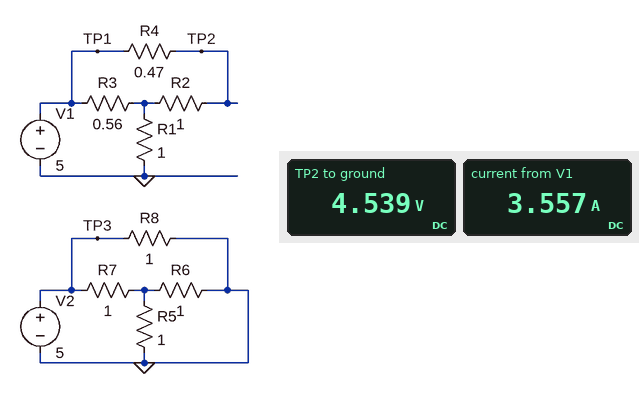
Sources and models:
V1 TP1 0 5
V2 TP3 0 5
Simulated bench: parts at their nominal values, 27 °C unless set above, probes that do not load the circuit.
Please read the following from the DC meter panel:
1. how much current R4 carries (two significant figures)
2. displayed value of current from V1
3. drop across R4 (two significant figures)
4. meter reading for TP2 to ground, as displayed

980 mA
3.557 A
460 mV
4.539 V
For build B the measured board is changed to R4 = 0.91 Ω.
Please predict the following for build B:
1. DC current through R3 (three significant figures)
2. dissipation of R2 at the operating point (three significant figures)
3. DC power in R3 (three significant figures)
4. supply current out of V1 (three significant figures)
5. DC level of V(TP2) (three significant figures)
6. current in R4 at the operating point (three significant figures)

2.70 A
626 mW
4.08 W
3.49 A
4.28 V
791 mA
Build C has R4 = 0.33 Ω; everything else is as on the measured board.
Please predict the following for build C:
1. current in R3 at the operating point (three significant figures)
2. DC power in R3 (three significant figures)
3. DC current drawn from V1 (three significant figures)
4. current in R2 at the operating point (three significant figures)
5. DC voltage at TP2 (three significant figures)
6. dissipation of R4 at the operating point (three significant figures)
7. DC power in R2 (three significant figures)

2.52 A
3.57 W
3.59 A
1.06 A
4.65 V
373 mW
1.13 W
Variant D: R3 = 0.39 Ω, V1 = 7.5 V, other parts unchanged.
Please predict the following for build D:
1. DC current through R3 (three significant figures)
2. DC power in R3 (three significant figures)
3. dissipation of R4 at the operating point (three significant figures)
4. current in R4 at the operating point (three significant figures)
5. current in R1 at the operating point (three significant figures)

4.53 A
8.01 W
679 mW
1.20 A
5.73 A
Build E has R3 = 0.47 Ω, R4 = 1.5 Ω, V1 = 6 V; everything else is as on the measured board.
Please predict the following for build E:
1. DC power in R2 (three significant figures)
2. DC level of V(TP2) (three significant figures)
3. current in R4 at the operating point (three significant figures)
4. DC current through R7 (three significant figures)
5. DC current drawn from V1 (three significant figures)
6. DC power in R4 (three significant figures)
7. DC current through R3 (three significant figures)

463 mW
4.98 V
680 mA
3.33 A
4.30 A
694 mW
3.62 A
